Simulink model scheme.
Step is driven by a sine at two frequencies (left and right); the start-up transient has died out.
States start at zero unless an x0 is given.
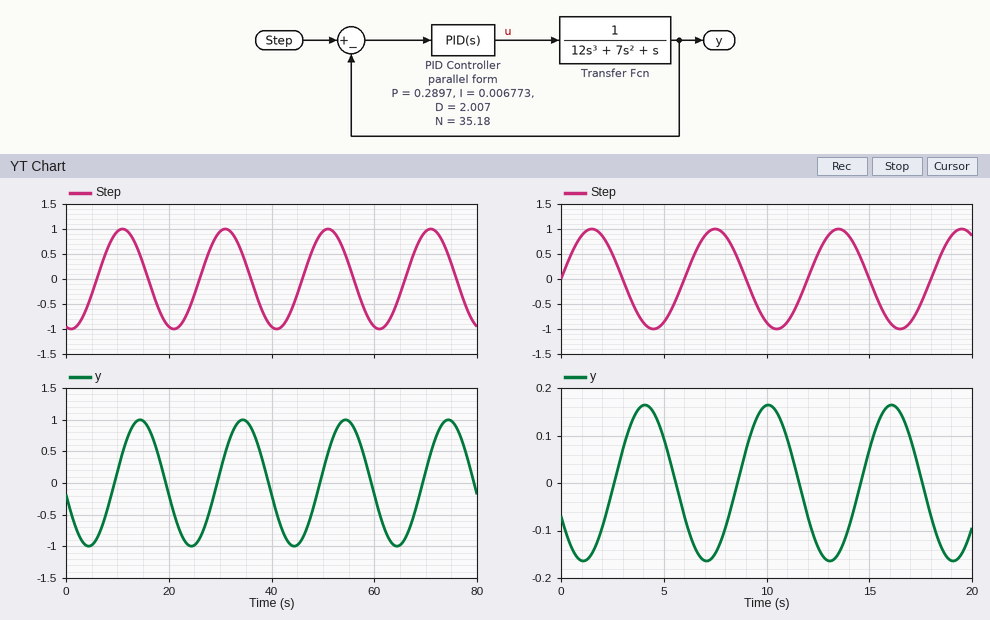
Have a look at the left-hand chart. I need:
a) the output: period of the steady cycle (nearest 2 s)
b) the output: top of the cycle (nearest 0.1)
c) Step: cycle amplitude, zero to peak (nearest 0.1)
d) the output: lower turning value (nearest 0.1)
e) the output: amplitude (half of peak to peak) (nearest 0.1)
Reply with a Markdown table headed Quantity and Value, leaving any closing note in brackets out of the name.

| Quantity | Value |
|---|---|
| the output: period of the steady cycle | 20 s |
| the output: top of the cycle | 1.0 |
| Step: cycle amplitude, zero to peak | 1.0 |
| the output: lower turning value | -1.0 |
| the output: amplitude (half of peak to peak) | 1.0 |
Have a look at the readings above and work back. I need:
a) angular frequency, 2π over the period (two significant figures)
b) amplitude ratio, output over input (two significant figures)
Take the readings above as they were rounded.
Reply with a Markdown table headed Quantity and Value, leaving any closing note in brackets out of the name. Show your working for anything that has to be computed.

| Quantity | Value |
|---|---|
| angular frequency, 2π over the period | 2π / 20 = 0.31 rad/s |
| amplitude ratio, output over input | 1 / 1 = 1.0 |
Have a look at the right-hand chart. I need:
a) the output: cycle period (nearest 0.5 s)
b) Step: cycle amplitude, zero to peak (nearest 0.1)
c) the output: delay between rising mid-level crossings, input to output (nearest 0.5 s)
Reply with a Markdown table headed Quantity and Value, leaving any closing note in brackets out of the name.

| Quantity | Value |
|---|---|
| the output: cycle period | 6.0 s |
| Step: cycle amplitude, zero to peak | 1.0 |
| the output: delay between rising mid-level crossings, input to output | 2.5 s |
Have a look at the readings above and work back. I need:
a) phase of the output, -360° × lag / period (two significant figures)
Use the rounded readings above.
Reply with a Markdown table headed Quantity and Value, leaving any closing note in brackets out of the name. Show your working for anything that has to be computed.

| Quantity | Value |
|---|---|
| phase of the output, -360° × lag / period | -360 × 2.5 / 6 = -150° |
